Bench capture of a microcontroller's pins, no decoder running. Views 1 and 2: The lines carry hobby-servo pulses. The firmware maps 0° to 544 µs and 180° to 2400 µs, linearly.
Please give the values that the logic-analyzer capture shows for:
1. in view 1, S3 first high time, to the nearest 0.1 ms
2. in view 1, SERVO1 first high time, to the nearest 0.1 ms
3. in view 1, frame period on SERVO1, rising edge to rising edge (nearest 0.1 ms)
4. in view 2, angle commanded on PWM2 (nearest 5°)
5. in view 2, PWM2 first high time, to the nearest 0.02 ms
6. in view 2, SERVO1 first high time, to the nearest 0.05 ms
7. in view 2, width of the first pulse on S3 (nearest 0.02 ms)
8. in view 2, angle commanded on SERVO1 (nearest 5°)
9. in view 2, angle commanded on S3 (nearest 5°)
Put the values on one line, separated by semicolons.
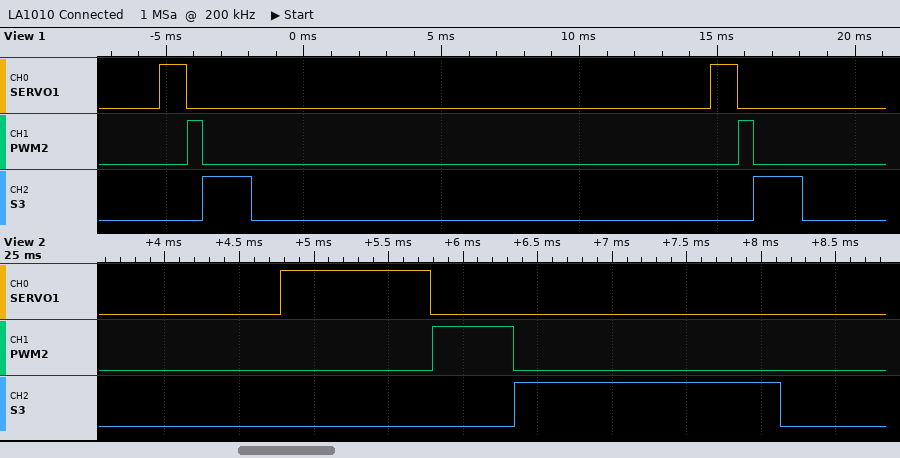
1.8 ms; 1.0 ms; 20.0 ms; 0°; 0.54 ms; 1.00 ms; 1.78 ms; 45°; 120°
